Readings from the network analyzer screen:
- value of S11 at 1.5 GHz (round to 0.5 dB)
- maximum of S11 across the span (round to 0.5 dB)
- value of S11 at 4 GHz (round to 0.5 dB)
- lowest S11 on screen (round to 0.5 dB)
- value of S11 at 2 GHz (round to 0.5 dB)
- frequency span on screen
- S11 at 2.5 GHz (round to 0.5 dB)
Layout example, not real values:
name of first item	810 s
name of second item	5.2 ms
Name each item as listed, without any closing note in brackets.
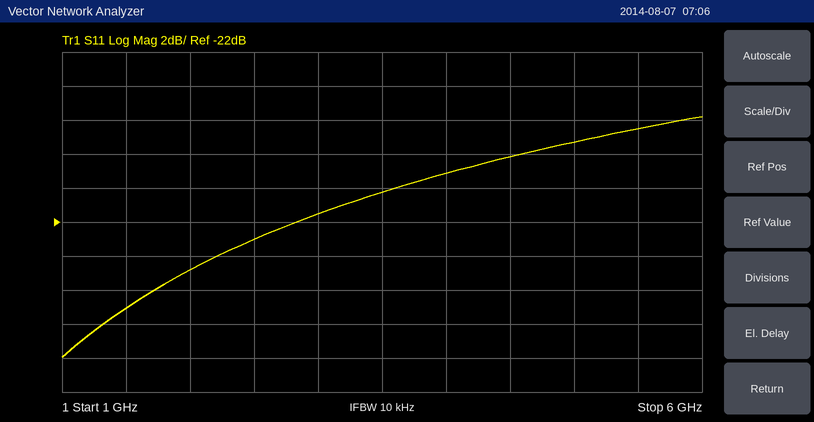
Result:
value of S11 at 1.5 GHz	-27.0 dB
maximum of S11 across the span	-16.0 dB
value of S11 at 4 GHz	-19.0 dB
lowest S11 on screen	-30.0 dB
value of S11 at 2 GHz	-25.0 dB
frequency span on screen	5 GHz
S11 at 2.5 GHz	-23.0 dB
